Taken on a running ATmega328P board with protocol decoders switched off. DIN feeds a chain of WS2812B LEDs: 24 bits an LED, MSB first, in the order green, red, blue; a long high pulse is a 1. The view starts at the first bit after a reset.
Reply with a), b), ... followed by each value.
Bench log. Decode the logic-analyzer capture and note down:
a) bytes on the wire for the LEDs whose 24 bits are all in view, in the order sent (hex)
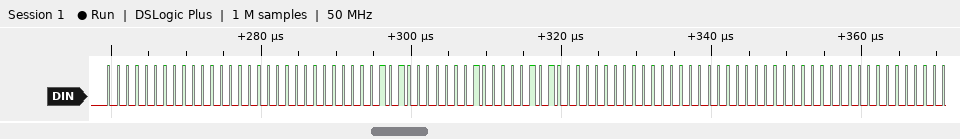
a) 00 00 00 05 01 05 00 00 00
